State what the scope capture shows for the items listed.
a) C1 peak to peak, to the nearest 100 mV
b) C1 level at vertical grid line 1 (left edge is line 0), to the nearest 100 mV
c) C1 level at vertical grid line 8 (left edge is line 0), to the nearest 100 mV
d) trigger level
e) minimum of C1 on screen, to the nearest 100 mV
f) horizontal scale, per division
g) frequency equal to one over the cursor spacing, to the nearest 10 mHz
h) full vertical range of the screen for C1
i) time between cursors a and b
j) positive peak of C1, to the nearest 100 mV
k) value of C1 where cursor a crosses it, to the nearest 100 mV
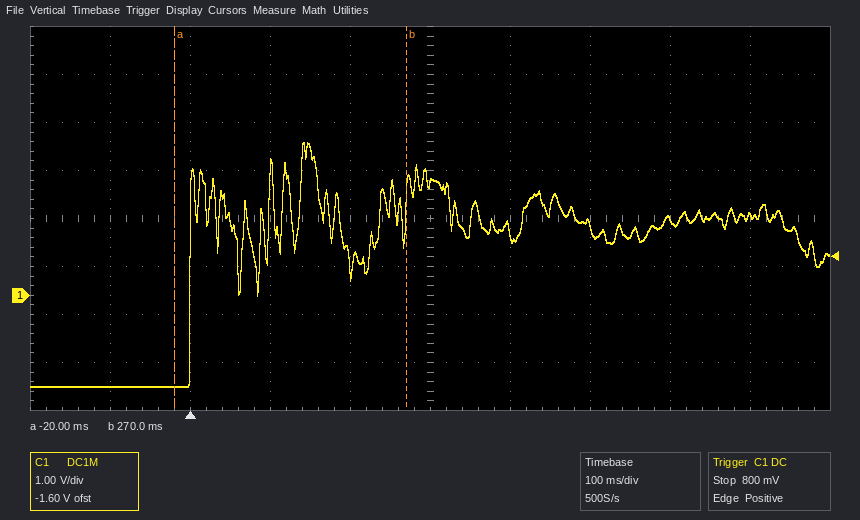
5.1 V
-1.9 V
1.6 V
800 mV
-1.9 V
100 ms
3.45 Hz
8 V
290 ms
3.2 V
-1.9 V
